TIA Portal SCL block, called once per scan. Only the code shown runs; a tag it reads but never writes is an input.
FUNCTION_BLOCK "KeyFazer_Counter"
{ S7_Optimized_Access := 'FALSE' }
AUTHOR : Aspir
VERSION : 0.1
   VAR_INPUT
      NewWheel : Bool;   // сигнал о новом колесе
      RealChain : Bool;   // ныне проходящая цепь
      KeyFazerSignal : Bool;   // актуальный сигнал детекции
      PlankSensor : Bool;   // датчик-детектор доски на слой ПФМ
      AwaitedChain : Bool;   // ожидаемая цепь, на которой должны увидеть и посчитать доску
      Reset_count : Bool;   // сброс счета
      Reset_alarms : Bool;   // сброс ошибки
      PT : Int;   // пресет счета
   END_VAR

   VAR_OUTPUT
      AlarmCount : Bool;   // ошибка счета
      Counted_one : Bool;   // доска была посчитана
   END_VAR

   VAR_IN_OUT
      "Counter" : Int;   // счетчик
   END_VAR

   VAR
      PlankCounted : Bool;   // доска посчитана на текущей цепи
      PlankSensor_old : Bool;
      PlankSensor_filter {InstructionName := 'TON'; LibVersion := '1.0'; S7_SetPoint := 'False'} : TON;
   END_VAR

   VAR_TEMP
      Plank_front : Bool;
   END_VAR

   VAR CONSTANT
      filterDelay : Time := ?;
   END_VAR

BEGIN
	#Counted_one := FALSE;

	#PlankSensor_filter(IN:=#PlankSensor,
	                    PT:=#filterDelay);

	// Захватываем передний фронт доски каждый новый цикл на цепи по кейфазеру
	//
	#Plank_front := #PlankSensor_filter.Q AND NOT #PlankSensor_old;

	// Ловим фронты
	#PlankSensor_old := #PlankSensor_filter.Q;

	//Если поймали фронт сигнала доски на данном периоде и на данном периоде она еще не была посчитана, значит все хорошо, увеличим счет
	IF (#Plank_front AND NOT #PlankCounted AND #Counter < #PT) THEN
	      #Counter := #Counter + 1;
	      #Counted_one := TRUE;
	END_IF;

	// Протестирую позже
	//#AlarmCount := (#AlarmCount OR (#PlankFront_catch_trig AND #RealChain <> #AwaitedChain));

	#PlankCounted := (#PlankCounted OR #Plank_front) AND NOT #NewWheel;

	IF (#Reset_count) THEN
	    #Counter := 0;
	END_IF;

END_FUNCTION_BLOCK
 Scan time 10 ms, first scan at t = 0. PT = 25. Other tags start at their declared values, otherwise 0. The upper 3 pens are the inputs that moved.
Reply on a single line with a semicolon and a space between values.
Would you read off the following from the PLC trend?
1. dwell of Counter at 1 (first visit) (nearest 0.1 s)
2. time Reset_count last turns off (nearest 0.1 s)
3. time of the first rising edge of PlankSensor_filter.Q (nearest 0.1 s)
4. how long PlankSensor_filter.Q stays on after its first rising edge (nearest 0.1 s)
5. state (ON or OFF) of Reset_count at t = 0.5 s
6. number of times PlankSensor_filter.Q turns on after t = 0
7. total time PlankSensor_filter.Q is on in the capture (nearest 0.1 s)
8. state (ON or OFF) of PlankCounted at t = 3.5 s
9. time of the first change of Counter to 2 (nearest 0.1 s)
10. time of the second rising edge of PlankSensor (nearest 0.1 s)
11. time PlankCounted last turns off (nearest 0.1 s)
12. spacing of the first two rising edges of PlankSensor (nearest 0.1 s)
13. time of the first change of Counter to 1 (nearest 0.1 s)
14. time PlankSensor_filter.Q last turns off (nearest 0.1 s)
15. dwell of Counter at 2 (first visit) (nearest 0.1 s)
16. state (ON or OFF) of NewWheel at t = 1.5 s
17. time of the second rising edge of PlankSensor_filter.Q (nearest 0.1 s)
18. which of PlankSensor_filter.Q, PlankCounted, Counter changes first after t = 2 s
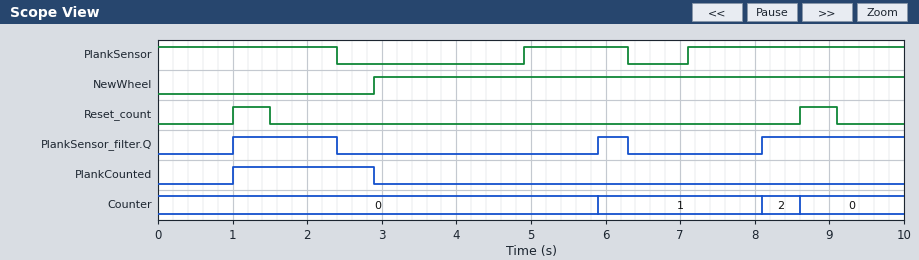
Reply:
2.2 s; 9.1 s; 1.0 s; 1.4 s; OFF; 3; 3.7 s; OFF; 8.1 s; 7.1 s; 2.9 s; 2.2 s; 5.9 s; 6.3 s; 0.5 s; OFF; 5.9 s; PlankSensor_filter.Q
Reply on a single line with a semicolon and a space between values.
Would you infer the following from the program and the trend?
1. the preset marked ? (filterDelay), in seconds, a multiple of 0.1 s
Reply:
1.0 s
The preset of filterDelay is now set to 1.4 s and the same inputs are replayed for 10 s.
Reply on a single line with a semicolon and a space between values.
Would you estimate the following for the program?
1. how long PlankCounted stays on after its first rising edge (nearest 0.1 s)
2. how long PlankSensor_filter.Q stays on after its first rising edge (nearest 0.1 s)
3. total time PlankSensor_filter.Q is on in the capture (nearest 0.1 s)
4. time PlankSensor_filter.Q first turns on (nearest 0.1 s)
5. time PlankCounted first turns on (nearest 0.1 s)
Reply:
1.5 s; 1.0 s; 2.5 s; 1.4 s; 1.4 s
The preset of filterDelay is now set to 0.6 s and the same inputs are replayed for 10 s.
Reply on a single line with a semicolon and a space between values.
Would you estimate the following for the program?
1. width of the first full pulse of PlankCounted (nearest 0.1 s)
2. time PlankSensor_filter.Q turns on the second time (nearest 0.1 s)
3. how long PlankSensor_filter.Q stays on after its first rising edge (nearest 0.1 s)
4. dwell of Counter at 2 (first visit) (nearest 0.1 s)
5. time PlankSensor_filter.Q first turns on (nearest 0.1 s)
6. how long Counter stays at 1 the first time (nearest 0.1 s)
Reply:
2.3 s; 5.5 s; 1.8 s; 0.9 s; 0.6 s; 0.4 s
